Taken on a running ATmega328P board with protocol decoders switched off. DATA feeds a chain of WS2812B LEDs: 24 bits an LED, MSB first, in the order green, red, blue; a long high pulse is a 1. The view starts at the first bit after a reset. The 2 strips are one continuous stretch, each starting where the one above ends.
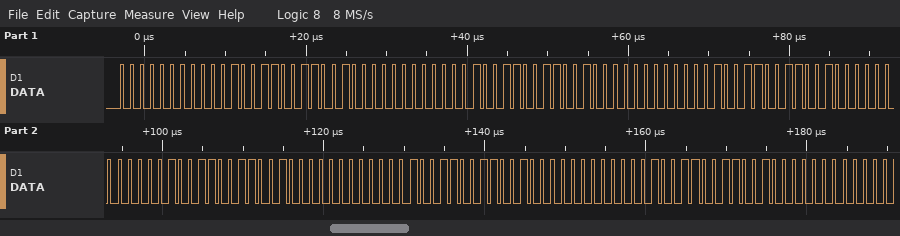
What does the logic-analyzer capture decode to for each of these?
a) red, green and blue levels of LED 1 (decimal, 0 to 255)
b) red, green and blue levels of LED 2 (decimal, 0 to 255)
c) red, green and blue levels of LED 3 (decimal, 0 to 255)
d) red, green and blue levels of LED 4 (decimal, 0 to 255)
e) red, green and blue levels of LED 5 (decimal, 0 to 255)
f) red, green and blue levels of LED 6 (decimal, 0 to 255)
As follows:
19, 0, 50
19, 0, 50
19, 0, 50
19, 0, 50
19, 0, 50
19, 0, 50
